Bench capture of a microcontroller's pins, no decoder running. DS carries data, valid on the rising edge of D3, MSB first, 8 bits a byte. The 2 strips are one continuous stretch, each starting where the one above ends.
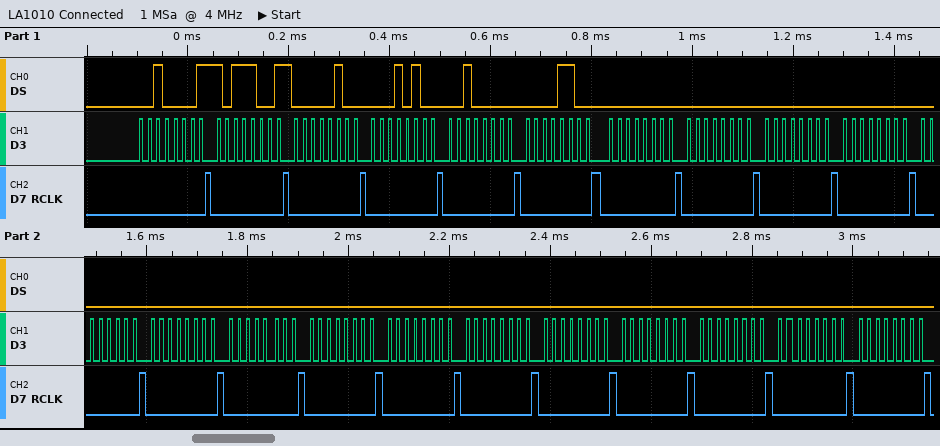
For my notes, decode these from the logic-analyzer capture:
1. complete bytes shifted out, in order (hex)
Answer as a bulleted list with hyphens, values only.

- 0x21 0xB9 0x04 0x14 0x20 0x0C 0x00 0x00 0x00 0x00 0x00 0x00 0x00 0x00 0x00 0x00 0x00 0x00 0x00 0x00 0x00
